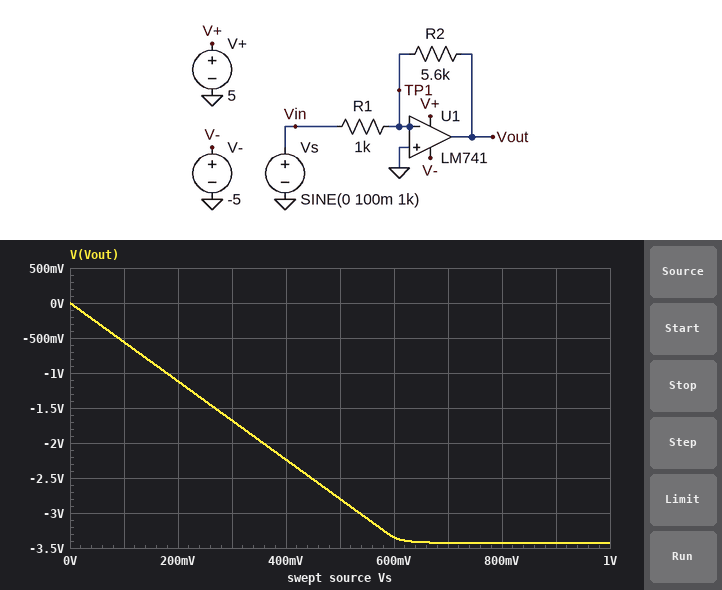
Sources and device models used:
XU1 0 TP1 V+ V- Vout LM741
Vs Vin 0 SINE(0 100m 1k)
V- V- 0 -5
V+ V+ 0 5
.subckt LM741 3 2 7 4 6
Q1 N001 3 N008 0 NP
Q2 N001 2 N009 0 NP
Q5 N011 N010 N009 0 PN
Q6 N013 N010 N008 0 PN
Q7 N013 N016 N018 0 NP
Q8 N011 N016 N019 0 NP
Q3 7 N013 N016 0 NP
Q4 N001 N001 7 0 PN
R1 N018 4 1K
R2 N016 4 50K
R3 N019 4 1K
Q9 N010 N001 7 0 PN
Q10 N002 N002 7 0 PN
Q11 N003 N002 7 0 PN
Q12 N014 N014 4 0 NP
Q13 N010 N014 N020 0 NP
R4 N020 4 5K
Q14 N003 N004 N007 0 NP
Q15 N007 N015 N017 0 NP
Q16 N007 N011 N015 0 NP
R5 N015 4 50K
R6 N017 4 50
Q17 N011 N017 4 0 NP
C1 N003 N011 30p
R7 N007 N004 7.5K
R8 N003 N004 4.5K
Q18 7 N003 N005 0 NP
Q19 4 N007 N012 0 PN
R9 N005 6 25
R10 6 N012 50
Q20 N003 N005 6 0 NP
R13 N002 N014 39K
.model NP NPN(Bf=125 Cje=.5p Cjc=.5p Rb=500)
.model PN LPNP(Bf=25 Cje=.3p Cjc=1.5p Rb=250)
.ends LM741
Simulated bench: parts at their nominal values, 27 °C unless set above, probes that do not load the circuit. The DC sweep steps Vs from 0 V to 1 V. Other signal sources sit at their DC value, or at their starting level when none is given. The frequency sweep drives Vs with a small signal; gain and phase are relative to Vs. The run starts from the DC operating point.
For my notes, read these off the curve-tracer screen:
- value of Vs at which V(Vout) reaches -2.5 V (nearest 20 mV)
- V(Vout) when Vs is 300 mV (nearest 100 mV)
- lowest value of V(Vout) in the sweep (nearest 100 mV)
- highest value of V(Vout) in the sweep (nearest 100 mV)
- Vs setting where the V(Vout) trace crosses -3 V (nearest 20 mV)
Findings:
440 mV
-1.7 V
-3.4 V
0 V
540 mV
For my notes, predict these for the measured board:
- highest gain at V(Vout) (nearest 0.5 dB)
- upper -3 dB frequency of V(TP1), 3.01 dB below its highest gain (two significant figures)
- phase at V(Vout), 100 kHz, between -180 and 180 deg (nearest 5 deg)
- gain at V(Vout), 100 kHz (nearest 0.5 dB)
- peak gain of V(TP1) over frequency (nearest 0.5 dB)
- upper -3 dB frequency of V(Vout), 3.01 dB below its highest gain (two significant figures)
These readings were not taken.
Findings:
15.0 dB
180 MHz
70 deg
3.0 dB
-0.5 dB
22 kHz
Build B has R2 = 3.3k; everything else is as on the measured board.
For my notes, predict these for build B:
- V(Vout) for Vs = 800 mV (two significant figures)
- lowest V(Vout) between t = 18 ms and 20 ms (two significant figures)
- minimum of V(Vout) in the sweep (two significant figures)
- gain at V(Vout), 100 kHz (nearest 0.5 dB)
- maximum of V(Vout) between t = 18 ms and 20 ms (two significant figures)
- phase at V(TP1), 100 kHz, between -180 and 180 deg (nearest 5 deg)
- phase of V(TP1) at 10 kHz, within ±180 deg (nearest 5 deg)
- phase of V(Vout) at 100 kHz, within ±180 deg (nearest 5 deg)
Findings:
-2.6 V
-330 mV
-3.3 V
1.0 dB
330 mV
15 deg
65 deg
55 deg
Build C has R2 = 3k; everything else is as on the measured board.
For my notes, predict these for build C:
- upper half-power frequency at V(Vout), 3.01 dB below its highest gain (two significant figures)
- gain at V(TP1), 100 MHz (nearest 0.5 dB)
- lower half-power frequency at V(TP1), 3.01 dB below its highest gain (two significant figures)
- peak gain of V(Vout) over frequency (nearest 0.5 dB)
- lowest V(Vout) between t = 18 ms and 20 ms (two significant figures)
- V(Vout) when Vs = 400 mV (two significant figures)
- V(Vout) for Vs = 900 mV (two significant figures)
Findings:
25 kHz
-3.0 dB
23 kHz
9.5 dB
-300 mV
-1.2 V
-2.7 V
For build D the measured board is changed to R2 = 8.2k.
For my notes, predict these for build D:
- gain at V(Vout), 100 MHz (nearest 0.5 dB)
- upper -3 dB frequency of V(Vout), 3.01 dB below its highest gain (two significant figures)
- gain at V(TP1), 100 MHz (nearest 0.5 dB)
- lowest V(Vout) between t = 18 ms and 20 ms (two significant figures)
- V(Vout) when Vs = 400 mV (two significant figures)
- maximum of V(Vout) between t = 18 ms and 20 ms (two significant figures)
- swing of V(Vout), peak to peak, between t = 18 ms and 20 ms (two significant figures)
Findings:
-18.5 dB
20 kHz
-2.0 dB
-820 mV
-3.3 V
820 mV
1.6 V
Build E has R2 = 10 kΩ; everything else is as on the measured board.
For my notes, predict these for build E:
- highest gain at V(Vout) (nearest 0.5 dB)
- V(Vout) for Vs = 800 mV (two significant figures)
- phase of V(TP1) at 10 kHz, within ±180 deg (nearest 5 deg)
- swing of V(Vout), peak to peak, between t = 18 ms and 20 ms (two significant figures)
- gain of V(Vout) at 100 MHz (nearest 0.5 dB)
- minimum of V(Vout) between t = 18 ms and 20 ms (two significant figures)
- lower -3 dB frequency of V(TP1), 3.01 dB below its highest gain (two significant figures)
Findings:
20.0 dB
-3.5 V
60 deg
2.0 V
-20.0 dB
-1.0 V
19 kHz
